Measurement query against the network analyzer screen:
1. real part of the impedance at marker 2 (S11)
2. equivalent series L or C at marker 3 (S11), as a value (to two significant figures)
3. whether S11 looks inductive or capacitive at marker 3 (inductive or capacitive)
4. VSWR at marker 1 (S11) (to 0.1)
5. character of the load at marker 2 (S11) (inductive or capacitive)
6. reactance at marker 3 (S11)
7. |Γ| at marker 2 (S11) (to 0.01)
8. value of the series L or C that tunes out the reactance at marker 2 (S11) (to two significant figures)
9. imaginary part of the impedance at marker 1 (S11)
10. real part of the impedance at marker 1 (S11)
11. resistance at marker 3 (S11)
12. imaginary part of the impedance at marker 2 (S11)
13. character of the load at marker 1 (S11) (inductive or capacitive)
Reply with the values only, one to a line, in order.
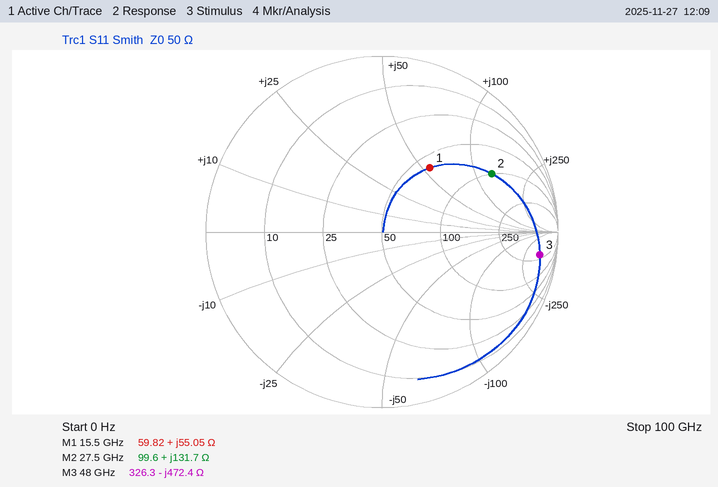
99.6 Ω
7.0 fF
capacitive
2.7
inductive
-472.4 Ω
0.71
44 fF
+55.05 Ω
59.82 Ω
326.3 Ω
+131.7 Ω
inductive
